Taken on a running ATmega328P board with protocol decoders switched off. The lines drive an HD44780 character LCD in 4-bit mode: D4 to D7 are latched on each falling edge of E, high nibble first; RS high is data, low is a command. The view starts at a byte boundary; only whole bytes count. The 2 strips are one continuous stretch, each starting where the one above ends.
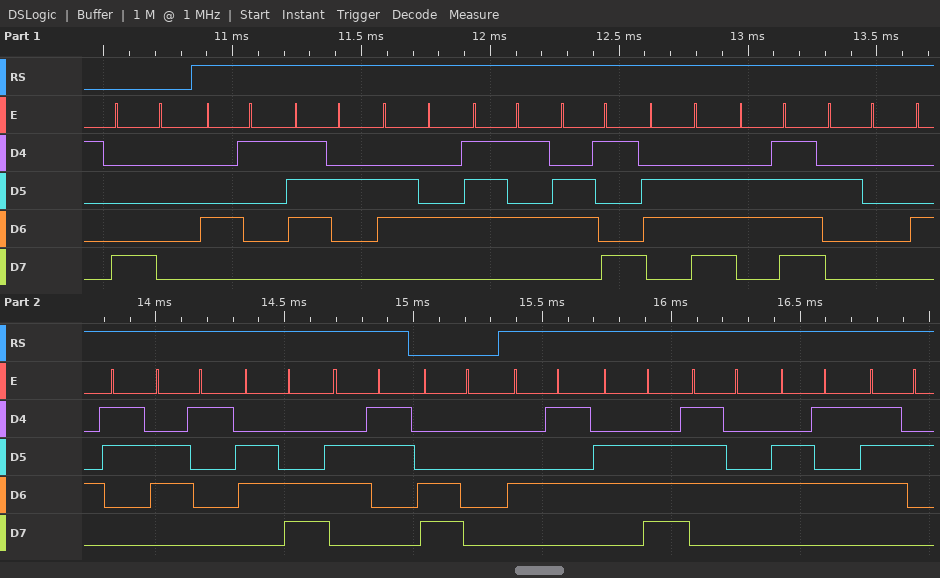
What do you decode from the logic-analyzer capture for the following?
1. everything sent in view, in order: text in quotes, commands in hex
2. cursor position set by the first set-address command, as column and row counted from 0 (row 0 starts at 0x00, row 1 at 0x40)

0x80 "Arduino Calc" 0xC0 "Enter"
column 0, row 0
